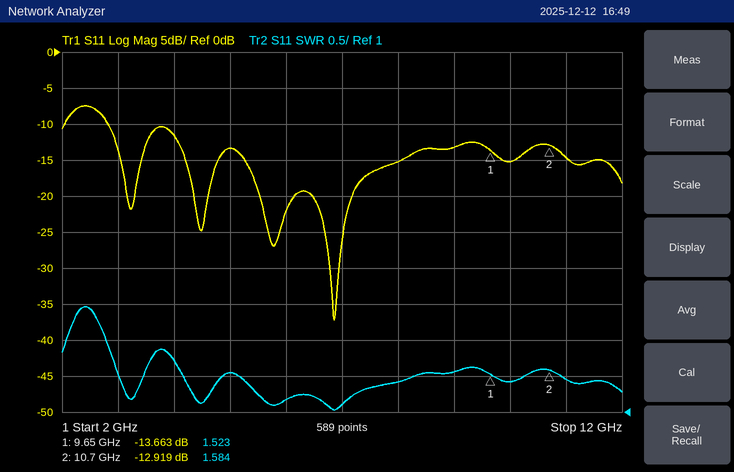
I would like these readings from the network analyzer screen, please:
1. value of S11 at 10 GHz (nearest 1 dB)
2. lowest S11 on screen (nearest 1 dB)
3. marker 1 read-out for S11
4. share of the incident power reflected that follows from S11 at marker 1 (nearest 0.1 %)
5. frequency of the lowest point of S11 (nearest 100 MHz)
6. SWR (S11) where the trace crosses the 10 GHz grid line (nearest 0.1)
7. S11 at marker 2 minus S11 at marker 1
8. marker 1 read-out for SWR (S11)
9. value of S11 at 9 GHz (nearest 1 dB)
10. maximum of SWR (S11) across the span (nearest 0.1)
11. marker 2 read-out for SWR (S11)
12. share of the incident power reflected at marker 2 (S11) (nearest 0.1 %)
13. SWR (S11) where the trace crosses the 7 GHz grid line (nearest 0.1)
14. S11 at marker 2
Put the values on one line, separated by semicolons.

-15 dB; -37 dB; -13.663 dB; 4.3 %; 6.9 GHz; 1.4; 0.744 dB; 1.523; -13 dB; 2.5; 1.584; 5.1 %; 1.1; -12.919 dB
